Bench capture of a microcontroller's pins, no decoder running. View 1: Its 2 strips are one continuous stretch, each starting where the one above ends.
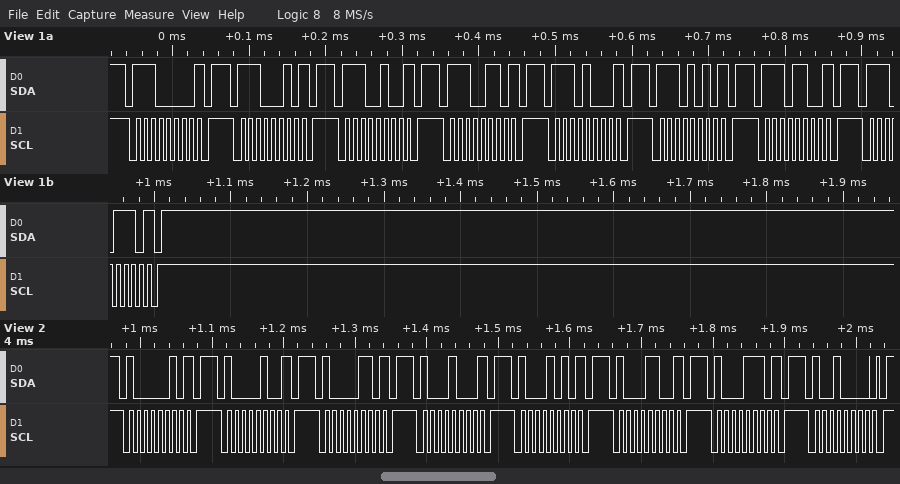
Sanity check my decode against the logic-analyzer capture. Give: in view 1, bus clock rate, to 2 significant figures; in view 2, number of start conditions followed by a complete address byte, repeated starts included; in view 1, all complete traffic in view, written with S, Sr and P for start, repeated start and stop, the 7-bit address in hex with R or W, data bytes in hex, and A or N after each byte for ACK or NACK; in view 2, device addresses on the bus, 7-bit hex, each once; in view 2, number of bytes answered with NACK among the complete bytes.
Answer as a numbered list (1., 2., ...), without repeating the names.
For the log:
1. 100 kHz
2. 8
3. S 70W N P S 71W N P S 72W N P S 73W N P S 74W N P S 75W N P S 76W N P S 77W N P
4. 0x41 0x42 0x43 0x44 0x45 0x46 0x47 0x48
5. 7
